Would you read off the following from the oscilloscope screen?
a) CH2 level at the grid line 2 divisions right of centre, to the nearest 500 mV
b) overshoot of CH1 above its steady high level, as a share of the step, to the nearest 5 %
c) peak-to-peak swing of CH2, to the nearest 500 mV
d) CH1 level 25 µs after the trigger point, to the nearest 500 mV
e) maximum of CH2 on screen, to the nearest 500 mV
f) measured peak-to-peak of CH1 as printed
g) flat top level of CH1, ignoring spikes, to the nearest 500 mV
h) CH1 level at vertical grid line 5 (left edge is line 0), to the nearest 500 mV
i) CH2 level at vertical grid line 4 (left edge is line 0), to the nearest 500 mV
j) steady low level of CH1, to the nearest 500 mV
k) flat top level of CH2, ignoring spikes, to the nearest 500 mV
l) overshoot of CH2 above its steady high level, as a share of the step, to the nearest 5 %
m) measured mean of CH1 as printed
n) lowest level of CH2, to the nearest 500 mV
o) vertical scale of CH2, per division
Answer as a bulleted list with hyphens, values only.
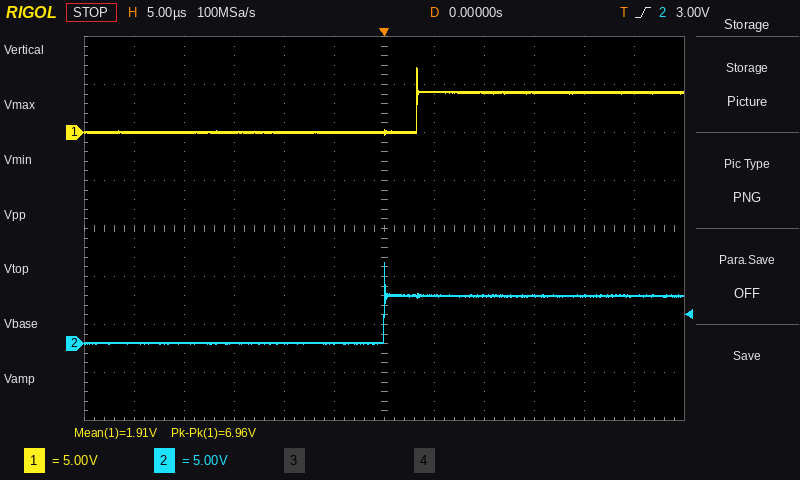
- 5.0 V
- 60 %
- 8.5 V
- 4.0 V
- 8.5 V
- 6.96 V
- 4.0 V
- 0.0 V
- 0.0 V
- 0.0 V
- 5.0 V
- 70 %
- 1.91 V
- 0.0 V
- 5 V
